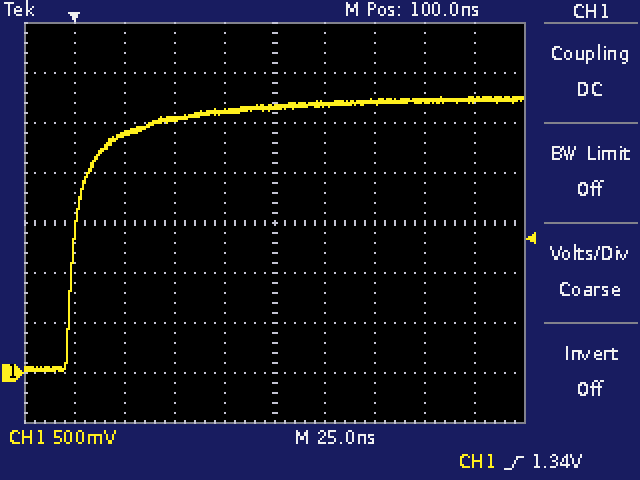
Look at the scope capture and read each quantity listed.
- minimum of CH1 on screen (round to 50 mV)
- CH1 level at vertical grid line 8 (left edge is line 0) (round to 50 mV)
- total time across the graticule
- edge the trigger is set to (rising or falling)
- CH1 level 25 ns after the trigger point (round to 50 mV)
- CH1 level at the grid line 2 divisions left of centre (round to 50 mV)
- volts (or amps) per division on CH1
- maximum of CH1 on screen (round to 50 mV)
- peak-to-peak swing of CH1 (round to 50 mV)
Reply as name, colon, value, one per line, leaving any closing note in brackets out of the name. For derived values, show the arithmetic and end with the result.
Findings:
minimum of CH1 on screen: 0 mV
CH1 level at vertical grid line 8 (left edge is line 0): 2.70 V
total time across the graticule: 250 ns
edge the trigger is set to: rising
CH1 level 25 ns after the trigger point: 2.40 V
CH1 level at the grid line 2 divisions left of centre: 2.55 V
volts (or amps) per division on CH1: 500 mV
maximum of CH1 on screen: 2.75 V
peak-to-peak swing of CH1: 2.75 V − (0 mV) = 2.75 V
